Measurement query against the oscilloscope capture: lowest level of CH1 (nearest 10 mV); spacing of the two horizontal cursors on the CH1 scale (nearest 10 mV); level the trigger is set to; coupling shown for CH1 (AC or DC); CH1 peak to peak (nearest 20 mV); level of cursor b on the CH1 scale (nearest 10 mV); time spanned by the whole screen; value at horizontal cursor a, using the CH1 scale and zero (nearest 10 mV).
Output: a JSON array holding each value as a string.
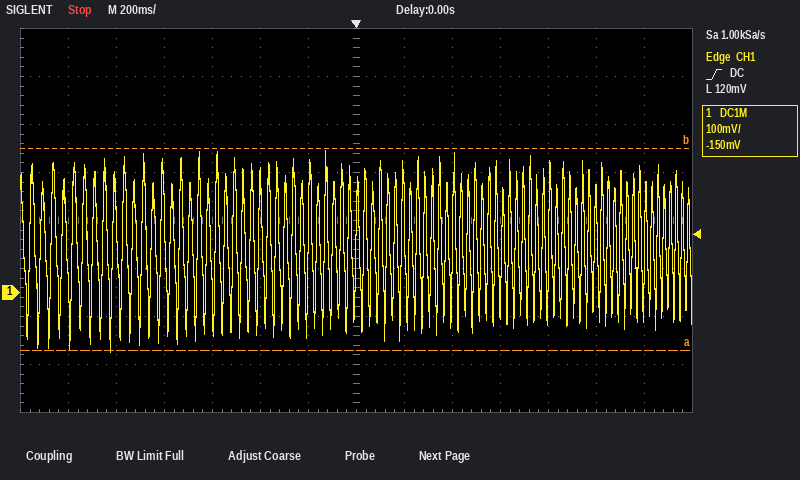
["-120 mV", "420 mV", "120 mV", "DC", "420 mV", "300 mV", "2.8 s", "-120 mV"]
